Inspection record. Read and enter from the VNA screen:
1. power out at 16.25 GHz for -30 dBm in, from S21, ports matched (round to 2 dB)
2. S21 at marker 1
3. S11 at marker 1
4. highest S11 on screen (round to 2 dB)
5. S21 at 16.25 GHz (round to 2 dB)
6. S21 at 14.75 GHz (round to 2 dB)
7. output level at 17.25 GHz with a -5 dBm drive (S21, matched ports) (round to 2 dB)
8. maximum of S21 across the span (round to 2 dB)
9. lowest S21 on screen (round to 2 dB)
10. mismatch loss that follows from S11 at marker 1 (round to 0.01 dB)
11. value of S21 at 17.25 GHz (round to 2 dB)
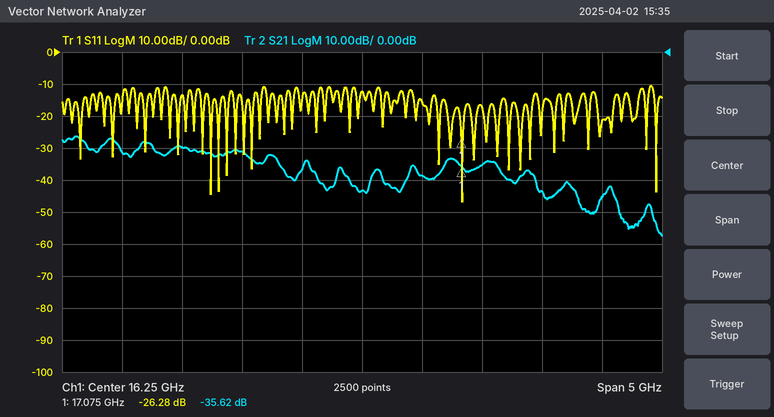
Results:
-74 dBm
-35.62 dB
-26.28 dB
-10 dB
-44 dB
-30 dB
-40 dBm
-26 dB
-58 dB
0.01 dB
-36 dB
